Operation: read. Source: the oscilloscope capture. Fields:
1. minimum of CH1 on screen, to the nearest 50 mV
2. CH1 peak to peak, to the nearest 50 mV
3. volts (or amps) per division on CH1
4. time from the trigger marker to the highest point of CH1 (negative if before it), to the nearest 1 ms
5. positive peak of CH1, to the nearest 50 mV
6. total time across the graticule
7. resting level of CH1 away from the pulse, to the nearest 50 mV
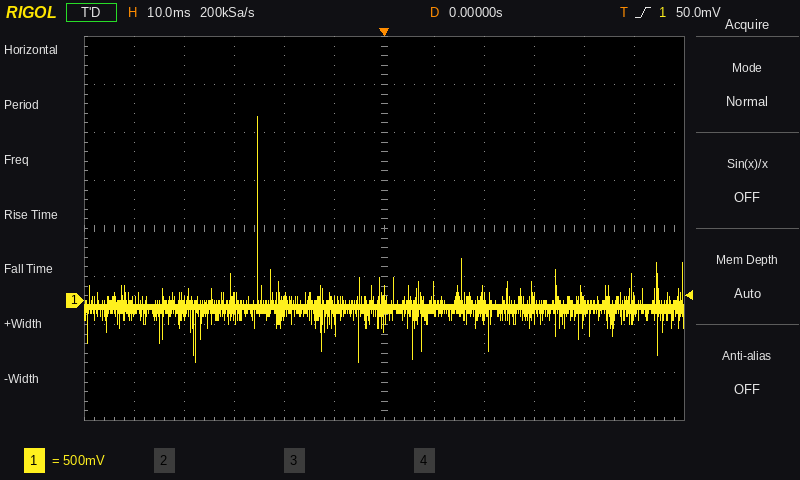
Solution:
-650 mV
2.55 V
500 mV
-25 ms
1.90 V
120 ms
-50 mV
